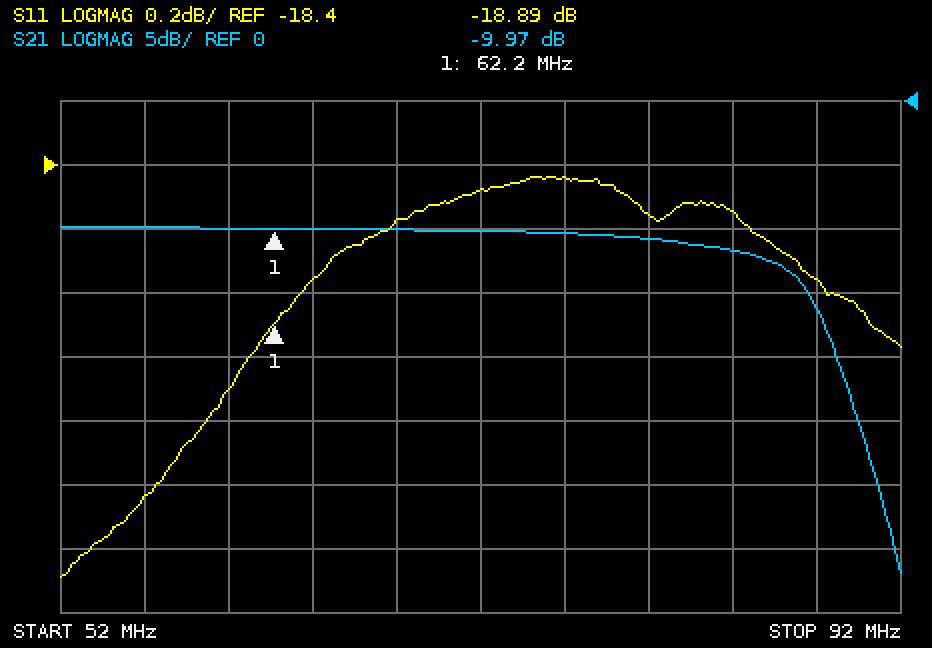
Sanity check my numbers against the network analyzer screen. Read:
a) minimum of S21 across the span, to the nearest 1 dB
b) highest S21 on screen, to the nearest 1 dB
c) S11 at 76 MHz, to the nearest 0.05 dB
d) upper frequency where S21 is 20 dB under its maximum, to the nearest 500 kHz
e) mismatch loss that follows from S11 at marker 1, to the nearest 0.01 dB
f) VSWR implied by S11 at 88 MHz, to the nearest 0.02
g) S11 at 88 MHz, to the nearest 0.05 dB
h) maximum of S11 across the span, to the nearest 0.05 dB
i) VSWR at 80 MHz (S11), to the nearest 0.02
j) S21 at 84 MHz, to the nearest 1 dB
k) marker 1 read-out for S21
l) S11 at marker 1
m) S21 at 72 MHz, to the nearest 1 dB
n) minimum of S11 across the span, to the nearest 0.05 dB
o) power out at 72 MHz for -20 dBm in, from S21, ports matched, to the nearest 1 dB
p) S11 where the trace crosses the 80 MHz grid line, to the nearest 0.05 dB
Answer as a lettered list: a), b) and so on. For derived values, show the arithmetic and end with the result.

a) -37 dB
b) -10 dB
c) -18.45 dB
d) 91.0 MHz
e) −10 log10(1 − 10^(-18.89/10)) ≈ 0.06 dB
f) |Γ| = 10^(-18.75/20) = 0.1155; VSWR = (1 + 0.1155)/(1 − 0.1155) ≈ 1.26
g) -18.75 dB
h) -18.45 dB
i) |Γ| = 10^(-18.55/20) = 0.1182; VSWR = (1 + 0.1182)/(1 − 0.1182) ≈ 1.27, so 1.26 to the nearest 0.02
j) -12 dB
k) -9.97 dB
l) -18.89 dB
m) -10 dB
n) -19.70 dB
o) -20 dBm + (-10 dB) = -30 dBm
p) -18.55 dB
